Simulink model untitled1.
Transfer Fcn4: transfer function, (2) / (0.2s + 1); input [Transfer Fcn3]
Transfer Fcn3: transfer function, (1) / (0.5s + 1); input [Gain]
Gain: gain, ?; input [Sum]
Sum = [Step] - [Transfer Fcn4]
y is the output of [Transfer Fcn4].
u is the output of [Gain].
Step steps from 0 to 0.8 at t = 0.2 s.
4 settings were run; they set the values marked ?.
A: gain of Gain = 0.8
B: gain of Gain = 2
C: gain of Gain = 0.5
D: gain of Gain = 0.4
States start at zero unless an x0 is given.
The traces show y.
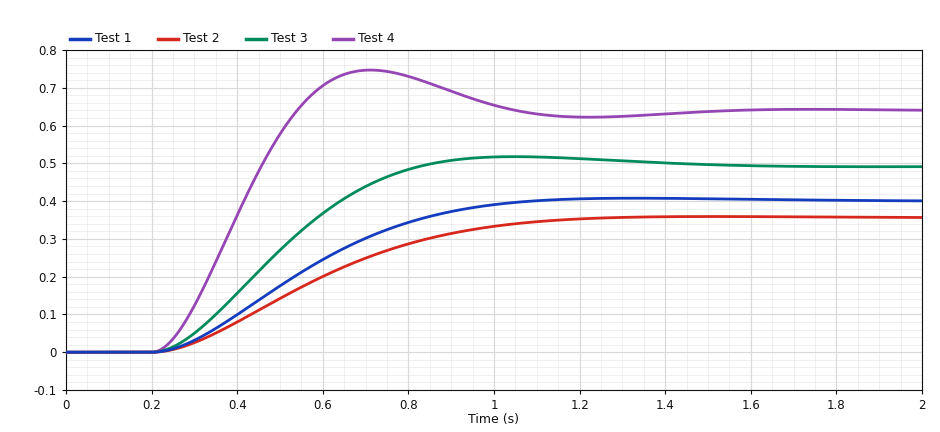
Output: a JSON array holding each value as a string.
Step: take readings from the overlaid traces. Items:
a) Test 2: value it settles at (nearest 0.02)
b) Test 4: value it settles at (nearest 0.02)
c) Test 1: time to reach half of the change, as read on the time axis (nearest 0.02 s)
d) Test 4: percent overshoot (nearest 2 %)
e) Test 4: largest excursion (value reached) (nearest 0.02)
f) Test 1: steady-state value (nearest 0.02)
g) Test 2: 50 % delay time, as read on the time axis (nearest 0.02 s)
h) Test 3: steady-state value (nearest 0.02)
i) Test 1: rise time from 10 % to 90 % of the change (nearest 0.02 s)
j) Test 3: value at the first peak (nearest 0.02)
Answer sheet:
["0.36", "0.64", "0.54 s", "16 %", "0.74", "0.40", "0.56 s", "0.50", "0.54 s", "0.52"]
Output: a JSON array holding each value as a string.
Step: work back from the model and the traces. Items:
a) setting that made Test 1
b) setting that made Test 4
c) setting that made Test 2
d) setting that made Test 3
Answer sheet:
["C", "B", "D", "A"]
